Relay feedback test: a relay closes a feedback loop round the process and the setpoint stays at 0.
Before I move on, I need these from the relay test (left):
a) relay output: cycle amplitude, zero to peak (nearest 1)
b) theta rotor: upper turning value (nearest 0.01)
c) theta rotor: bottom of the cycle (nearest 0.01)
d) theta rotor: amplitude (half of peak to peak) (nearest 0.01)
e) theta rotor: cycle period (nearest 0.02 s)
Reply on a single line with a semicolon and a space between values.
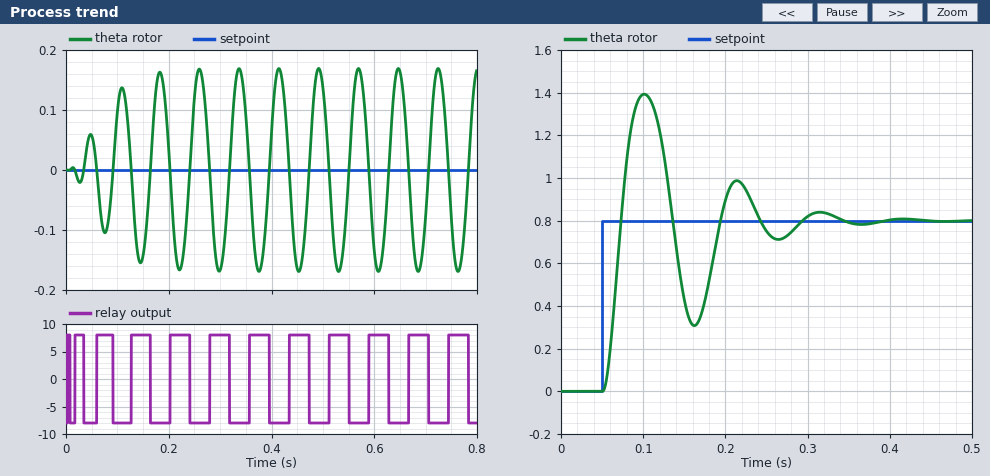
8; 0.17; -0.17; 0.17; 0.08 s
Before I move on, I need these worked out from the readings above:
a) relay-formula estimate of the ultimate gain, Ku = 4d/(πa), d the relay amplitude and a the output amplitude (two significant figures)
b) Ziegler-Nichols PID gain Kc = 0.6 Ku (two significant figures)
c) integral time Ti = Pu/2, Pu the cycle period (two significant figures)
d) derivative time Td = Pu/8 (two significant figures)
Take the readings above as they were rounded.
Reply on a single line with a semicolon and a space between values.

60; 36; 0.040 s; 0.010 s
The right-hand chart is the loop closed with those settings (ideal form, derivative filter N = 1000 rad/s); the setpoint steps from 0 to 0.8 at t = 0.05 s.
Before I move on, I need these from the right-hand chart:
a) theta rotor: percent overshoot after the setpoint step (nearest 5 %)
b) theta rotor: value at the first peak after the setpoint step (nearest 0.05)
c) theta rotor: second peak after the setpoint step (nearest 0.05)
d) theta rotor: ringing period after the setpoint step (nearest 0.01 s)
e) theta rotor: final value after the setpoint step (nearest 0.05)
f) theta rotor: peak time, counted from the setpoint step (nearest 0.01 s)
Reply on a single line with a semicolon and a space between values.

75 %; 1.40; 1.00; 0.11 s; 0.80; 0.05 s
